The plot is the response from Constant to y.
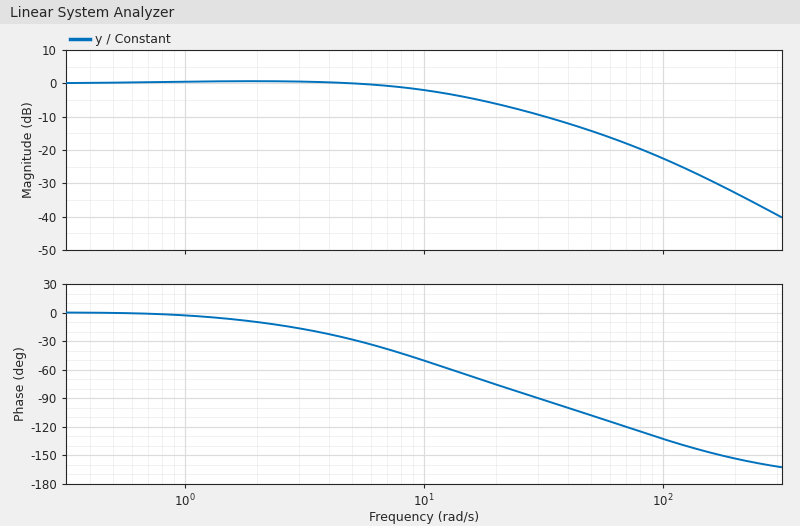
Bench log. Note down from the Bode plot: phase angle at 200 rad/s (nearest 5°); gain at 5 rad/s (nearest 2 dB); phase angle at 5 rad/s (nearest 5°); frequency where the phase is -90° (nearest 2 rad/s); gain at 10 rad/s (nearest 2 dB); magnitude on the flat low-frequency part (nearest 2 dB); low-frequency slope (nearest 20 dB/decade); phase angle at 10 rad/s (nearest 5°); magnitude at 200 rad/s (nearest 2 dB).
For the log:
-155°
0 dB
-30°
30 rad/s
-2 dB
0 dB
0 dB/decade
-50°
-32 dB
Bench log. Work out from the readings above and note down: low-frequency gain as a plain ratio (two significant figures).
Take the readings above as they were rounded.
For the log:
1.0
